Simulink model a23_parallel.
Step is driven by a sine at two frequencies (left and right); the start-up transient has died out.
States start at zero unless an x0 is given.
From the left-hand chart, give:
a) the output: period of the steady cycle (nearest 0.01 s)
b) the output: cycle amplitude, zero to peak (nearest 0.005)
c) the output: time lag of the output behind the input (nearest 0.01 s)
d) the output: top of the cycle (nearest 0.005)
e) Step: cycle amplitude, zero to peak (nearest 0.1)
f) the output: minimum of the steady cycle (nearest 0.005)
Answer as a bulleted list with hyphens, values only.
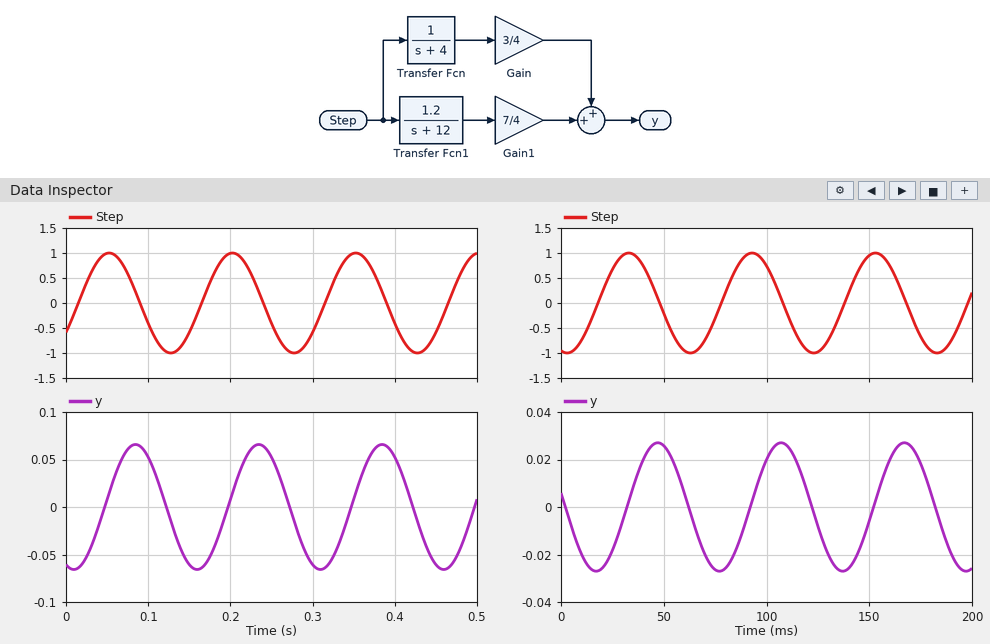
- 0.15 s
- 0.065
- 0.03 s
- 0.065
- 1.0
- -0.065
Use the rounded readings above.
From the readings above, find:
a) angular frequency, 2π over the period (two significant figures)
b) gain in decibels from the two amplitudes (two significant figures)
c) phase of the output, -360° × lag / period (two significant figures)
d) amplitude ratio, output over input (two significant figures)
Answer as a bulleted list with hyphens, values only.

- 42 rad/s
- -24 dB
- -72°
- 0.065
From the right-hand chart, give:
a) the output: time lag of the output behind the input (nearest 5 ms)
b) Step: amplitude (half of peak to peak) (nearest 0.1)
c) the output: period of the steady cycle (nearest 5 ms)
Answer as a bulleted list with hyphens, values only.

- 15 ms
- 1.0
- 60 ms
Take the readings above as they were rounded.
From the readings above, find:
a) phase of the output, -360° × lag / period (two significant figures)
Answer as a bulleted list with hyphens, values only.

- -90°
